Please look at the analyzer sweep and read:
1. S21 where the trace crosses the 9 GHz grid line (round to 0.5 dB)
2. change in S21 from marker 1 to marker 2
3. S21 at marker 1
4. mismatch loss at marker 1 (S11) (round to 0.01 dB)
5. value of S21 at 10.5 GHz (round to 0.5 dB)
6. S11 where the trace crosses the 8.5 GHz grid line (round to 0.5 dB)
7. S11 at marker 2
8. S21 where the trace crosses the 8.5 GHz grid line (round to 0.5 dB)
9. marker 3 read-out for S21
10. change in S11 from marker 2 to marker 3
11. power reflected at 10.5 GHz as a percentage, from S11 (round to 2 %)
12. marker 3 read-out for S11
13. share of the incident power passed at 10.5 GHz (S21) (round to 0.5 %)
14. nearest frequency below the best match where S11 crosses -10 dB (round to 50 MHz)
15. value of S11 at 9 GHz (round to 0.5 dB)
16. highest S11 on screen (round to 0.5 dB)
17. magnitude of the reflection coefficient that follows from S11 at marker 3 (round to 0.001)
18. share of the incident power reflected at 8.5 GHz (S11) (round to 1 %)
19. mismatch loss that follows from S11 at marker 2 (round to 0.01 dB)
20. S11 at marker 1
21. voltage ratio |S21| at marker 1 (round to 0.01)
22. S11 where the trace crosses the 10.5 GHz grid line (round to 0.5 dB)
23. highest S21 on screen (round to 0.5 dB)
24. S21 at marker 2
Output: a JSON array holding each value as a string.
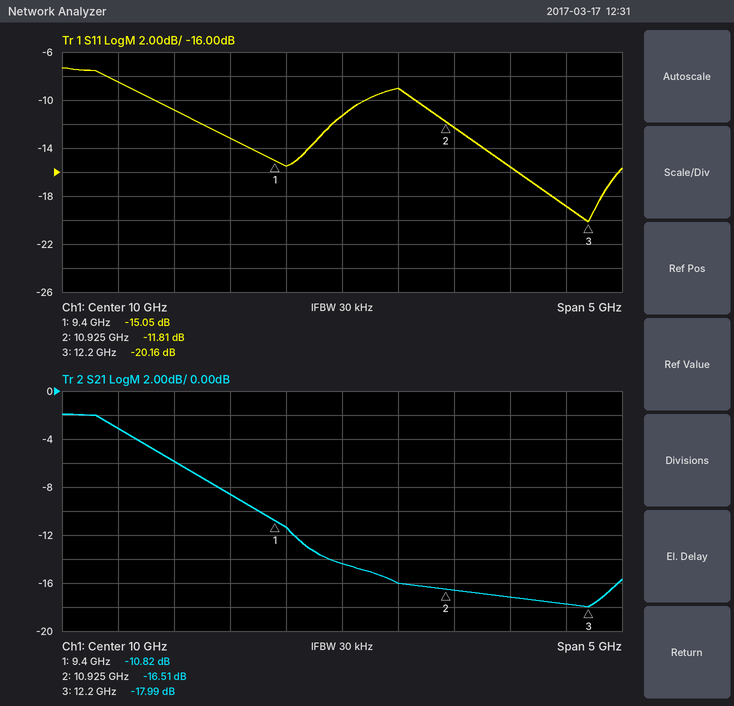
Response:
["-8.5 dB", "-5.69 dB", "-10.82 dB", "0.14 dB", "-16.0 dB", "-11.0 dB", "-11.81 dB", "-6.0 dB", "-17.99 dB", "-8.35 dB", "12 %", "-20.16 dB", "2.5 %", "10.65 GHz", "-13.0 dB", "-7.5 dB", "0.098", "8 %", "0.30 dB", "-15.05 dB", "0.29", "-9.0 dB", "-2.0 dB", "-16.51 dB"]
